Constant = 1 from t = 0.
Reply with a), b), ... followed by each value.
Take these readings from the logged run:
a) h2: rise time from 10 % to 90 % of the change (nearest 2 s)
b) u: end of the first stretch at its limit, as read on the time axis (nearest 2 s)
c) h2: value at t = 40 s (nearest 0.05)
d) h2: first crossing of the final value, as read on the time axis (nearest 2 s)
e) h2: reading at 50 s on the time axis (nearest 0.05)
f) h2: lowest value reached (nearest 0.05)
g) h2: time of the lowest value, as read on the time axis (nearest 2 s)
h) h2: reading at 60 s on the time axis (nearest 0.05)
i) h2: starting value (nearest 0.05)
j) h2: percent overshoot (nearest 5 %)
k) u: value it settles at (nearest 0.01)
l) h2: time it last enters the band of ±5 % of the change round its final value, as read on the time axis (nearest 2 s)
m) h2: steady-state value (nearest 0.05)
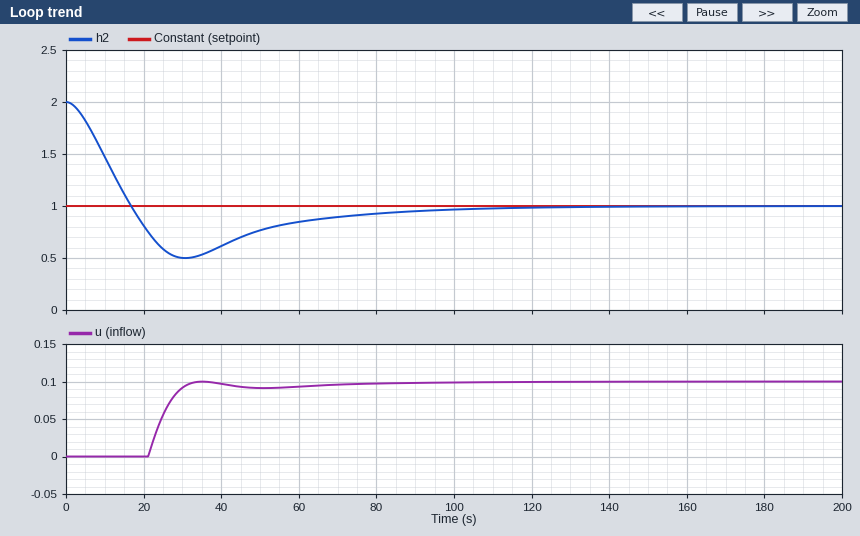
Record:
a) 12 s
b) 22 s
c) 0.60
d) 16 s
e) 0.75
f) 0.50
g) 30 s
h) 0.85
i) 2.00
j) 50 %
k) 0.10
l) 90 s
m) 1.00
